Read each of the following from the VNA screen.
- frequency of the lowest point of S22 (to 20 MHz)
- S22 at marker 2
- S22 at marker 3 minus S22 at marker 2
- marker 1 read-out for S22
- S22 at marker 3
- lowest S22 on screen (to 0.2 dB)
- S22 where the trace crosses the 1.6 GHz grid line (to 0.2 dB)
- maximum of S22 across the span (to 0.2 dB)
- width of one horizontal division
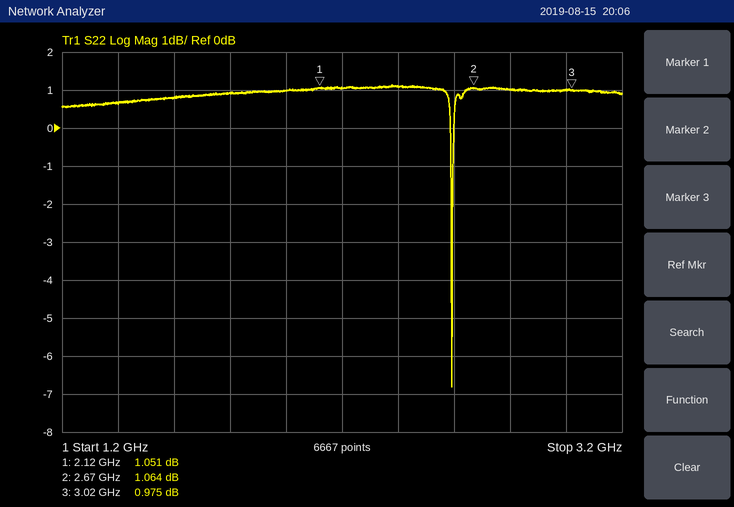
2.60 GHz
1.064 dB
-0.089 dB
1.051 dB
0.975 dB
-6.8 dB
0.8 dB
1.2 dB
200 MHz
